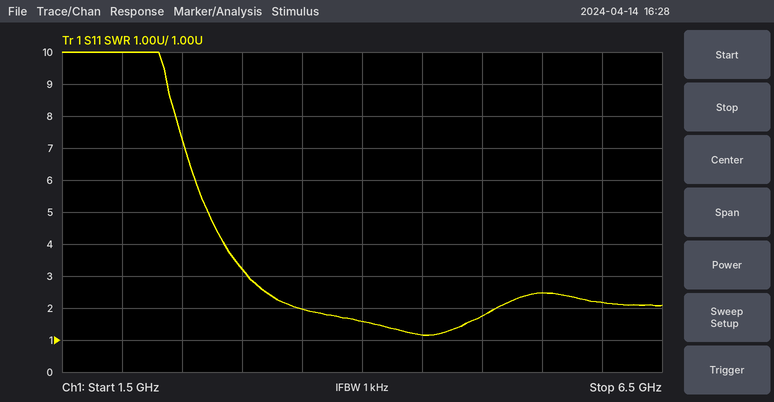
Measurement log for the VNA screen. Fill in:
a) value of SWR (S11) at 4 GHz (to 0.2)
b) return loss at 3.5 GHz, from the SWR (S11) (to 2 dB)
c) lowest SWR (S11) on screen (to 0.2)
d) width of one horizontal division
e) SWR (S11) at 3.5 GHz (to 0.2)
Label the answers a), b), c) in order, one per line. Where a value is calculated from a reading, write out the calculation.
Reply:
a) 1.6
b) −20 log10((2 − 1)/(2 + 1)) ≈ 10 dB
c) 1.2
d) 500 MHz
e) 2.0
